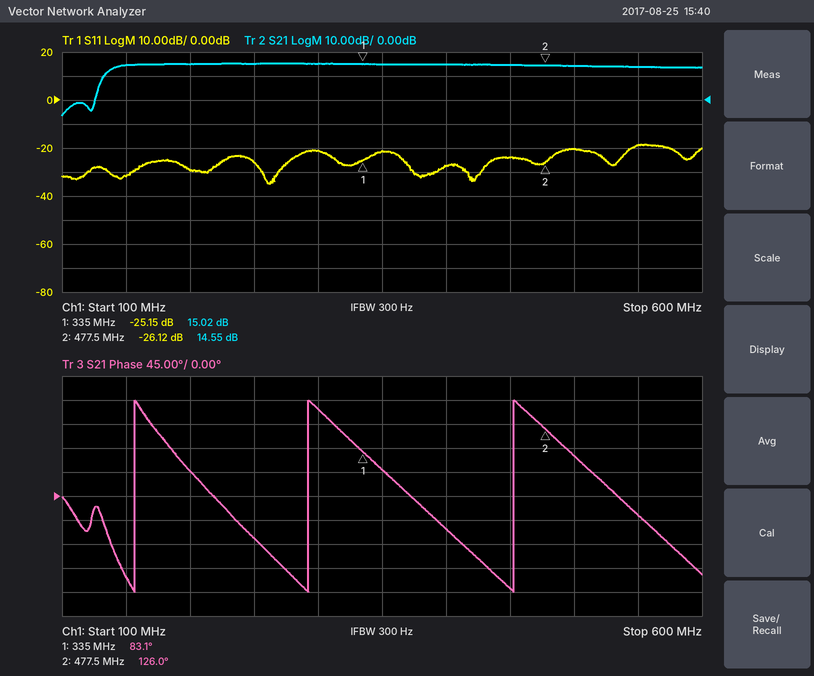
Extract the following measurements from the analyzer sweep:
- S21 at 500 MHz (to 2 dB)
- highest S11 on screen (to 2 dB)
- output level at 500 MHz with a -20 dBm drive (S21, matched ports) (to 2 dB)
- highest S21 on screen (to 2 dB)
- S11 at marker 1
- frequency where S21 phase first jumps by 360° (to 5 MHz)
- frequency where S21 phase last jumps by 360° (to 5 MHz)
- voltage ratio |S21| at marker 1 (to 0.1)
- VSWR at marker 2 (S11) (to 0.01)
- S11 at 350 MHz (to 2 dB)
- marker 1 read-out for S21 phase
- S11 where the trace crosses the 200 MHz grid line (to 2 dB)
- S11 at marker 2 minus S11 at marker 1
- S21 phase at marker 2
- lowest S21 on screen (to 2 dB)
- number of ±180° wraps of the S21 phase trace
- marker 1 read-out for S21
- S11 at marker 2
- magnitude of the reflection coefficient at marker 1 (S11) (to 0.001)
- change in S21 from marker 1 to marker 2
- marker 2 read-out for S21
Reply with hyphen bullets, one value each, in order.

- 14 dB
- -18 dB
- -6 dBm
- 16 dB
- -25.15 dB
- 155 MHz
- 455 MHz
- 5.6
- 1.10
- -22 dB
- 83.1°
- -30 dB
- -0.97 dB
- 126.0°
- -6 dB
- 3
- 15.02 dB
- -26.12 dB
- 0.055
- -0.47 dB
- 14.55 dB
